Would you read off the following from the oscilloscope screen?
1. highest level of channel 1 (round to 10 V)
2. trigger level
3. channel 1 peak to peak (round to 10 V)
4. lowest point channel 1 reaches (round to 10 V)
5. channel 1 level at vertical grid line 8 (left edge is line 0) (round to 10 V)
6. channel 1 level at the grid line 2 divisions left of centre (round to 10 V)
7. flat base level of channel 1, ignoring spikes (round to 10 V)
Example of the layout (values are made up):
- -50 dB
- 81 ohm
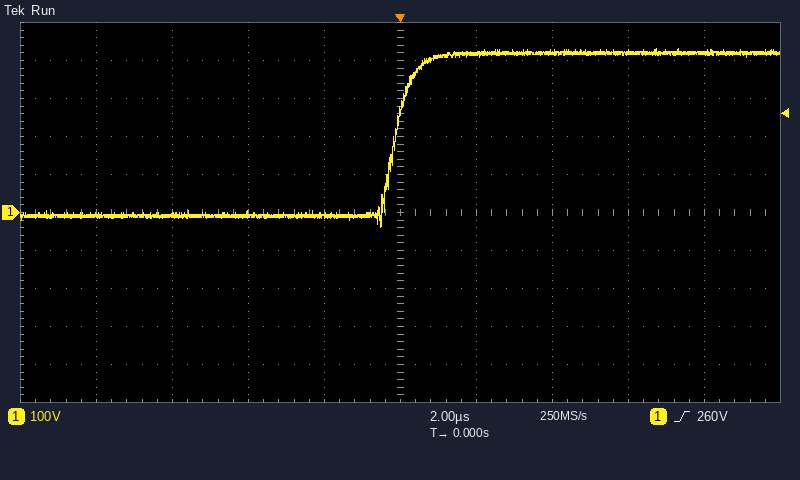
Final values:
- 430 V
- 260 V
- 470 V
- -40 V
- 420 V
- -10 V
- -10 V
